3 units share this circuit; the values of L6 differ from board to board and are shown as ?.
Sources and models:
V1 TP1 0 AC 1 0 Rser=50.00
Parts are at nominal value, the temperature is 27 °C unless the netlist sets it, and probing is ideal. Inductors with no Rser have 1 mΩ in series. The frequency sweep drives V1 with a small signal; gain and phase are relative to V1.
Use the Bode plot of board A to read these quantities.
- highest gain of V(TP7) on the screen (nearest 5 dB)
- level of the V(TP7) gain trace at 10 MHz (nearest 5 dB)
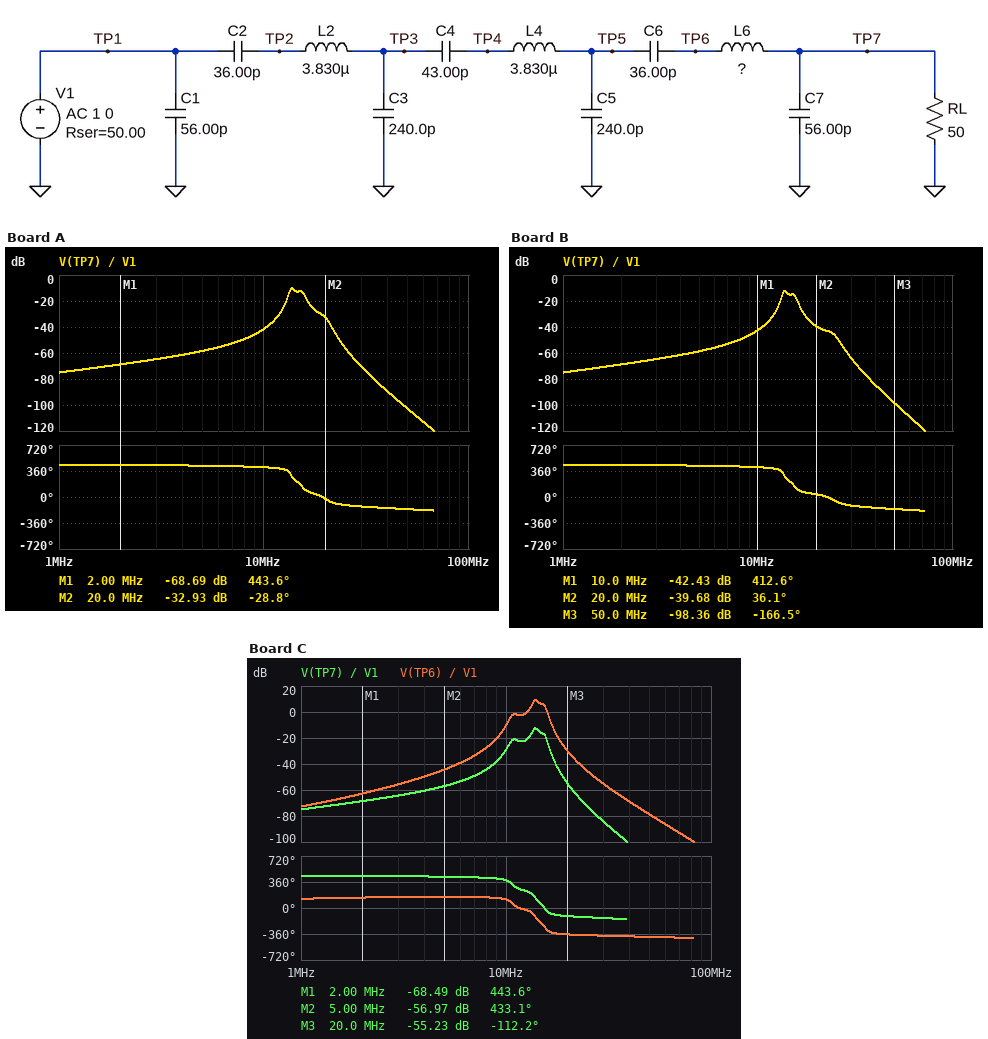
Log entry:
-10 dB
-40 dB
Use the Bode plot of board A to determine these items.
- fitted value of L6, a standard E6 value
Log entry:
2.2 µH
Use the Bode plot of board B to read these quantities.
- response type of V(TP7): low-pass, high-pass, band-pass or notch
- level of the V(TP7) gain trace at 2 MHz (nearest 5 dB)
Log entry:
band-pass
-70 dB
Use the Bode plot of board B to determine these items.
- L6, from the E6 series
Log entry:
1.5 µH
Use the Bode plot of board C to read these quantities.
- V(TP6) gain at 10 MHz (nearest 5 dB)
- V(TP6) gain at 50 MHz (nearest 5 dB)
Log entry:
-10 dB
-80 dB
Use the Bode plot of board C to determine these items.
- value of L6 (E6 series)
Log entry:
6.8 µH
